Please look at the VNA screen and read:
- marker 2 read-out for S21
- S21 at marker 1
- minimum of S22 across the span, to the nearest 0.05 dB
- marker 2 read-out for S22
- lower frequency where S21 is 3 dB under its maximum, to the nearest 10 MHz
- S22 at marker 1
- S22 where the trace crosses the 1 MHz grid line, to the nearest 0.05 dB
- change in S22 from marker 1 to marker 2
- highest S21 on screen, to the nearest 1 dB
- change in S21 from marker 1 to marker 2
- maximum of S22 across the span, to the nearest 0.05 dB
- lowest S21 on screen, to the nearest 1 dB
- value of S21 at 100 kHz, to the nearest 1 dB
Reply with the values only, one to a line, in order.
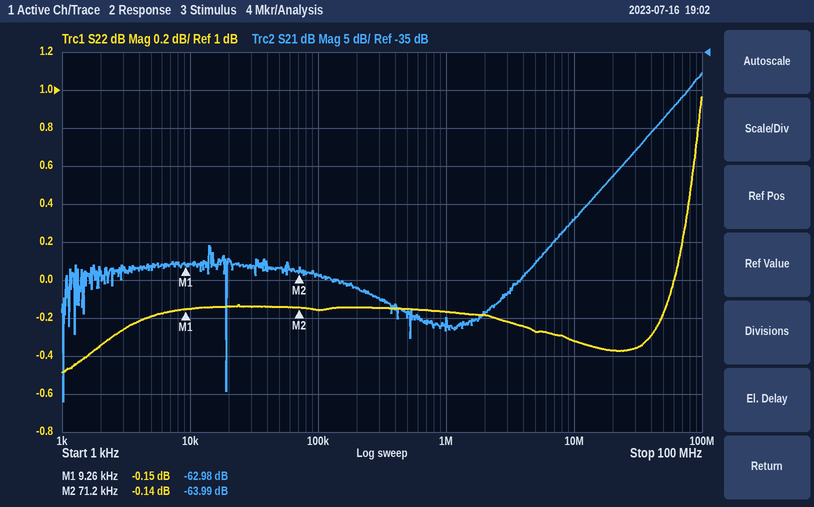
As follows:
-63.99 dB
-62.98 dB
-0.50 dB
-0.14 dB
70 MHz
-0.15 dB
-0.15 dB
0.01 dB
-38 dB
-1.01 dB
0.95 dB
-81 dB
-64 dB
